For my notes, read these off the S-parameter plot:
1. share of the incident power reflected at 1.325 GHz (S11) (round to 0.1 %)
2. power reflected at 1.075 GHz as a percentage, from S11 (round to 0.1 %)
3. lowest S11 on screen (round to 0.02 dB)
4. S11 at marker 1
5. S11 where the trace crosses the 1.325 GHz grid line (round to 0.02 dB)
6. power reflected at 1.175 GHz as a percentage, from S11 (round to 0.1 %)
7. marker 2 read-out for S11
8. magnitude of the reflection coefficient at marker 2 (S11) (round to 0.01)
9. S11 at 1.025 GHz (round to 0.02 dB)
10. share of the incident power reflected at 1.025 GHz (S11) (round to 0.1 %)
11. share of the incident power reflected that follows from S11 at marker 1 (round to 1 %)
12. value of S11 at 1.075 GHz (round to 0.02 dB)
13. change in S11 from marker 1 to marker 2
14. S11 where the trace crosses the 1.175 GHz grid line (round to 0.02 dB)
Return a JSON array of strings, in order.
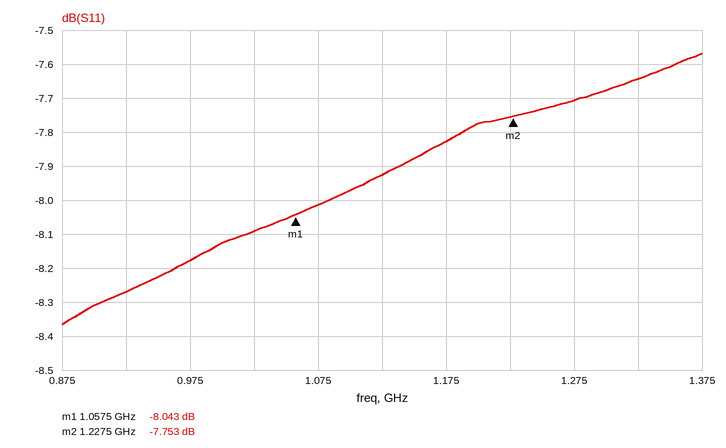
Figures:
["17.2 %", "15.8 %", "-8.36 dB", "-8.043 dB", "-7.64 dB", "16.5 %", "-7.753 dB", "0.41", "-8.10 dB", "15.5 %", "16 %", "-8.02 dB", "0.290 dB", "-7.82 dB"]
